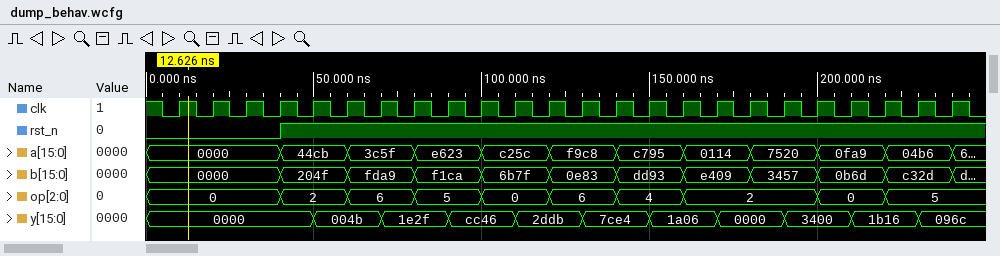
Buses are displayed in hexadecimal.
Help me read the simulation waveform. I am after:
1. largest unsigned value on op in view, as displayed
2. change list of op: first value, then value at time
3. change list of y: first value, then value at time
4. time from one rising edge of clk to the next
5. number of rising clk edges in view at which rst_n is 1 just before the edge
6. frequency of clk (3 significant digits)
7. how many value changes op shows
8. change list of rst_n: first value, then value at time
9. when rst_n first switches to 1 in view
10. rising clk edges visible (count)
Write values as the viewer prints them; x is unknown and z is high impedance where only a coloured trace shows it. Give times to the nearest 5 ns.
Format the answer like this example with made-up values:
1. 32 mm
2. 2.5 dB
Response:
1. 6
2. 0, 2 at 40 ns, 6 at 60 ns, 5 at 80 ns, 0 at 100 ns, 6 at 120 ns, 4 at 140 ns, 2 at 160 ns, 0 at 200 ns, 5 at 220 ns
3. 0000, 004b at 50 ns, 1e2f at 70 ns, cc46 at 90 ns, 2ddb at 110 ns, 7ce4 at 130 ns, 1a06 at 150 ns, 0000 at 170 ns, 3400 at 190 ns, 1b16 at 210 ns, 096c at 230 ns
4. 10 ns
5. 20
6. 100 MHz
7. 9
8. 0, 1 at 40 ns
9. 40 ns
10. 24
